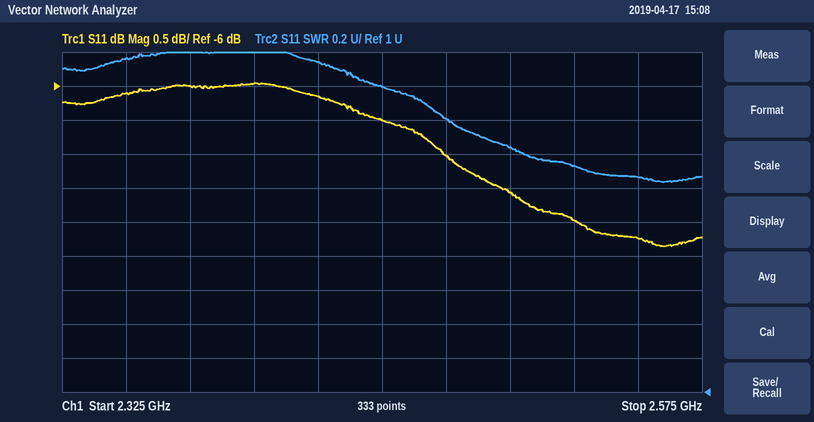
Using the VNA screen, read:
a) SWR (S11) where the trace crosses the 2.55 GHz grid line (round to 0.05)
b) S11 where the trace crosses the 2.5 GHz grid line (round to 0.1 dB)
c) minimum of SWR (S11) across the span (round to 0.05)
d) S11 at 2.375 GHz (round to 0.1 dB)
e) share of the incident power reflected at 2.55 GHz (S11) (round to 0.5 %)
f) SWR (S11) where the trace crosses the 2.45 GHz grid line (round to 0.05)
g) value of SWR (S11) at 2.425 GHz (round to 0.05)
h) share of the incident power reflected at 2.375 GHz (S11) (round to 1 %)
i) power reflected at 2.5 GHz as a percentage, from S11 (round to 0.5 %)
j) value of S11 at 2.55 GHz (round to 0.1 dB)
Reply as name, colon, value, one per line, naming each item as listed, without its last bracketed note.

SWR (S11) where the trace crosses the 2.55 GHz grid line: 2.25
S11 where the trace crosses the 2.5 GHz grid line: -7.6 dB
minimum of SWR (S11) across the span: 2.25
S11 at 2.375 GHz: -6.0 dB
share of the incident power reflected at 2.55 GHz (S11): 15.0 %
SWR (S11) where the trace crosses the 2.45 GHz grid line: 2.80
value of SWR (S11) at 2.425 GHz: 2.95
share of the incident power reflected at 2.375 GHz (S11): 25 %
power reflected at 2.5 GHz as a percentage, from S11: 17.5 %
value of S11 at 2.55 GHz: -8.2 dB
